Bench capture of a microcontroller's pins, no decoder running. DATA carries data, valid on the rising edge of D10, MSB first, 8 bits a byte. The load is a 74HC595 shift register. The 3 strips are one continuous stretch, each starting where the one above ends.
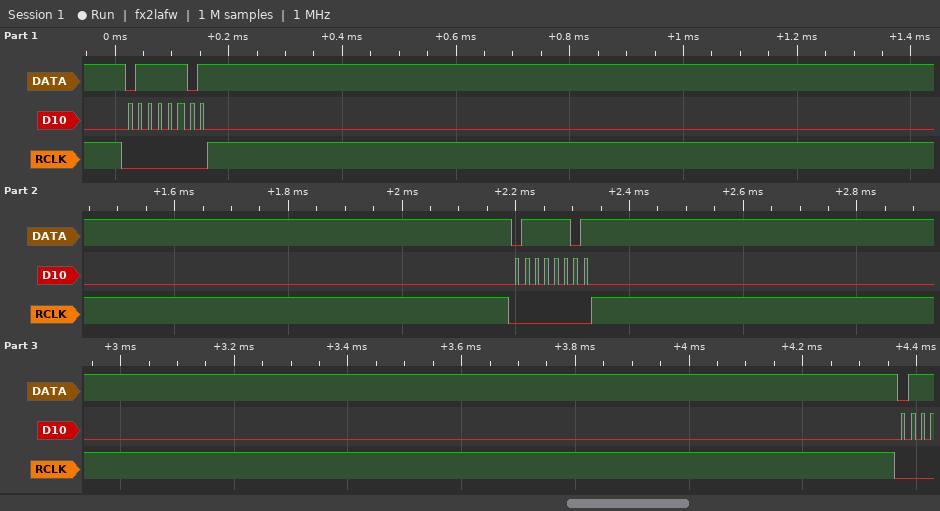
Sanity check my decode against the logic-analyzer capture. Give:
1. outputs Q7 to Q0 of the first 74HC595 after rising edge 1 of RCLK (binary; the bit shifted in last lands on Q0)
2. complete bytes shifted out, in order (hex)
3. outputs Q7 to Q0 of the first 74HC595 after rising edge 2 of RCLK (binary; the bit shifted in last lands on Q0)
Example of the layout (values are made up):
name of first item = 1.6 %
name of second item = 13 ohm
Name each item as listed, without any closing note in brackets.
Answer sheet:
outputs Q7 to Q0 of the first 74HC595 after rising edge 1 of RCLK = 01111101
complete bytes shifted out, in order = 0x7D 0x7D
outputs Q7 to Q0 of the first 74HC595 after rising edge 2 of RCLK = 01111101
